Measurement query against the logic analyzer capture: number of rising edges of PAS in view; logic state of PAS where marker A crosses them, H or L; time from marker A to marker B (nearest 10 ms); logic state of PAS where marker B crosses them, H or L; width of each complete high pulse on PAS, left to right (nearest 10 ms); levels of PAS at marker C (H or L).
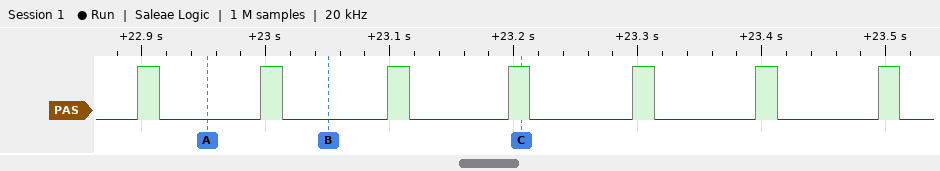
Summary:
7
PAS=L
100 ms
PAS=L
20 ms, 20 ms, 20 ms, 20 ms, 20 ms, 20 ms, 20 ms
PAS=H
